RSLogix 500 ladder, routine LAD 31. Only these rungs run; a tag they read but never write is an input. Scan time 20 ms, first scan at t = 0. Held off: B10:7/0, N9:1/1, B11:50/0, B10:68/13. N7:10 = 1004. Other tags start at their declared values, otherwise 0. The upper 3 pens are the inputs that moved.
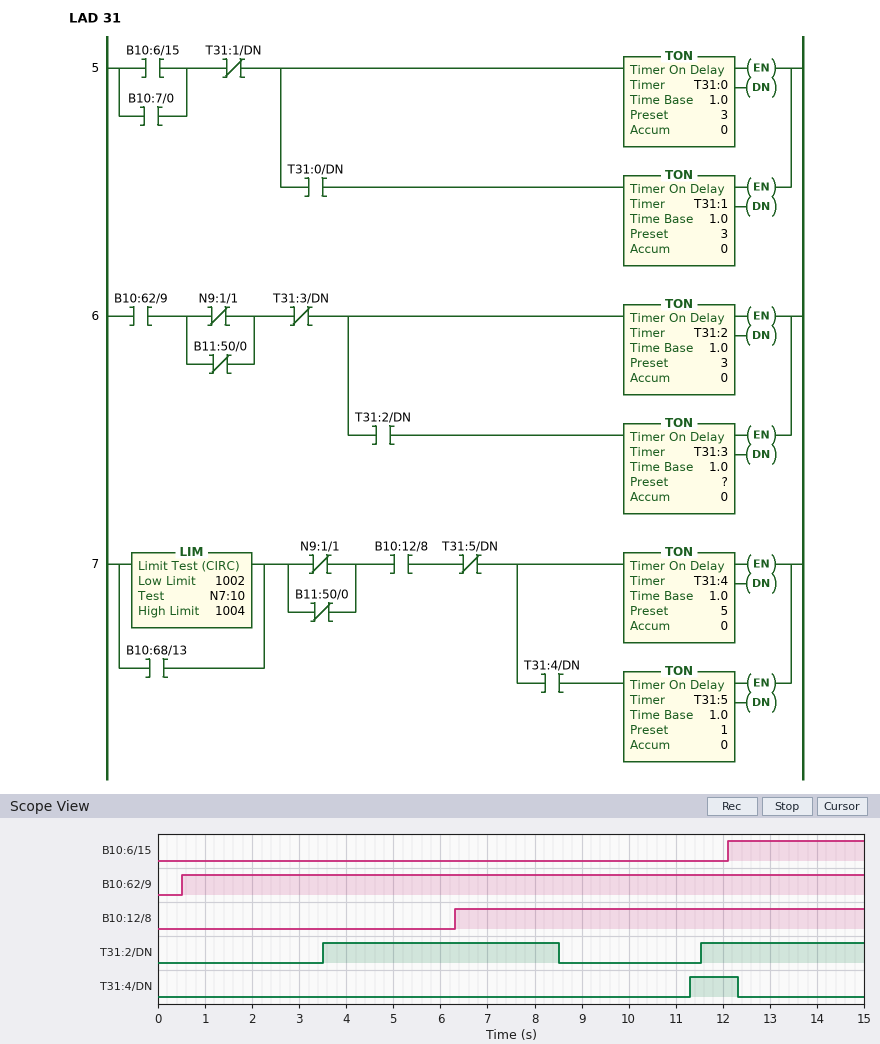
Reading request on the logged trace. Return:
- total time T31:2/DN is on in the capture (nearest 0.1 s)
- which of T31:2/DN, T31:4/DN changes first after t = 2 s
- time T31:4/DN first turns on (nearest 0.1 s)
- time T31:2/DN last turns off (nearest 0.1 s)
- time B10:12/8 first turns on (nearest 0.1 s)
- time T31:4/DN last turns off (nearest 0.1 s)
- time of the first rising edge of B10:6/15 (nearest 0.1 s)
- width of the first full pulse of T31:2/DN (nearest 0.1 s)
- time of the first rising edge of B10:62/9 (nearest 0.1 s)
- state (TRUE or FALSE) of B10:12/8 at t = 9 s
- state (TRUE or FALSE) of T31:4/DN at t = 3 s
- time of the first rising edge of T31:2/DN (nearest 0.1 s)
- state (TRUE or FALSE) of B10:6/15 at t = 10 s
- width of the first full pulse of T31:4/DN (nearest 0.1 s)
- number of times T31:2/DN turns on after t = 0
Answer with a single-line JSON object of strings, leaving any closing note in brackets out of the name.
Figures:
{"total time T31:2/DN is on in the capture": "8.5 s", "which of T31:2/DN, T31:4/DN changes first after t = 2 s": "T31:2/DN", "time T31:4/DN first turns on": "11.3 s", "time T31:2/DN last turns off": "8.5 s", "time B10:12/8 first turns on": "6.3 s", "time T31:4/DN last turns off": "12.3 s", "time of the first rising edge of B10:6/15": "12.1 s", "width of the first full pulse of T31:2/DN": "5.0 s", "time of the first rising edge of B10:62/9": "0.5 s", "state (TRUE or FALSE) of B10:12/8 at t = 9 s": "TRUE", "state (TRUE or FALSE) of T31:4/DN at t = 3 s": "FALSE", "time of the first rising edge of T31:2/DN": "3.5 s", "state (TRUE or FALSE) of B10:6/15 at t = 10 s": "FALSE", "width of the first full pulse of T31:4/DN": "1.0 s", "number of times T31:2/DN turns on after t = 0": "2"}
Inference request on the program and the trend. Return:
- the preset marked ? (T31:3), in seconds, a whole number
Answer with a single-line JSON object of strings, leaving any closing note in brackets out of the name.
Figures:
{"the preset marked ? (T31:3), in seconds, a whole number": "5 s"}
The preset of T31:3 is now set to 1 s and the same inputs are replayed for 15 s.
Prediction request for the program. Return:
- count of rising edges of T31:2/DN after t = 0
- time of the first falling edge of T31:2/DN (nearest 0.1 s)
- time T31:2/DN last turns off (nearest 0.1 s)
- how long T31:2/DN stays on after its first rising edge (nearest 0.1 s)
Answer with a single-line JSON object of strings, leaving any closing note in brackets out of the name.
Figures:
{"count of rising edges of T31:2/DN after t = 0": "3", "time of the first falling edge of T31:2/DN": "4.5 s", "time T31:2/DN last turns off": "12.6 s", "how long T31:2/DN stays on after its first rising edge": "1.0 s"}
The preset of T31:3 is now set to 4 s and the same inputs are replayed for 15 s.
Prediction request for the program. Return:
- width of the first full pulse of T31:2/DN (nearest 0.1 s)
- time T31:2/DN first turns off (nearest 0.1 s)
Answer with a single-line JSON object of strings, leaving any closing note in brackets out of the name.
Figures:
{"width of the first full pulse of T31:2/DN": "4.0 s", "time T31:2/DN first turns off": "7.5 s"}
